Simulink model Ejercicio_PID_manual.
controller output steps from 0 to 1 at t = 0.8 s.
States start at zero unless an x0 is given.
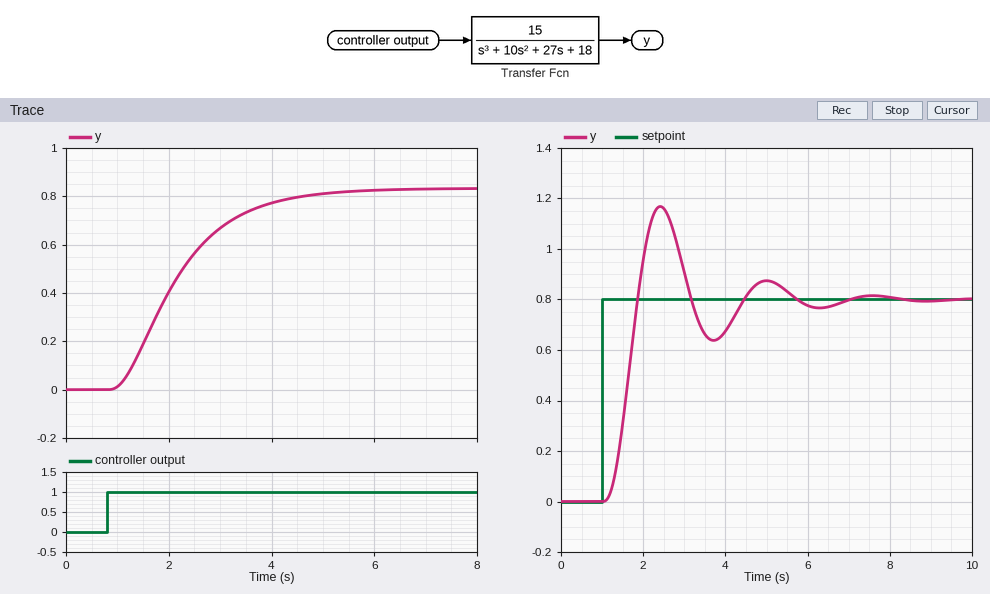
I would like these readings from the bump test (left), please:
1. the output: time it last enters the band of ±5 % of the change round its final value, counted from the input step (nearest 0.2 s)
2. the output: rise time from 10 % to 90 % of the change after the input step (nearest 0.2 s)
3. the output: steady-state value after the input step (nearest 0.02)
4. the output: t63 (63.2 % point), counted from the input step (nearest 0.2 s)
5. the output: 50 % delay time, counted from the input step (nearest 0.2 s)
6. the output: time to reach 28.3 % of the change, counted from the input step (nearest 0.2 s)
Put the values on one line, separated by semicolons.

3.6 s; 2.4 s; 0.84; 1.6 s; 1.2 s; 0.8 s
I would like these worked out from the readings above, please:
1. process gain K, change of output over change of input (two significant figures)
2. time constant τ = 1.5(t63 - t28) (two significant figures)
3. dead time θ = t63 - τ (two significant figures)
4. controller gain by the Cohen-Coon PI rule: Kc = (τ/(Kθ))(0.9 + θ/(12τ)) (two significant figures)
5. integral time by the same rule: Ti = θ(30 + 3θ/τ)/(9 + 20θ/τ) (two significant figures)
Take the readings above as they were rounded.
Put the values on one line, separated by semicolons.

0.84; 1.2 s; 0.40 s; 3.3; 0.79 s
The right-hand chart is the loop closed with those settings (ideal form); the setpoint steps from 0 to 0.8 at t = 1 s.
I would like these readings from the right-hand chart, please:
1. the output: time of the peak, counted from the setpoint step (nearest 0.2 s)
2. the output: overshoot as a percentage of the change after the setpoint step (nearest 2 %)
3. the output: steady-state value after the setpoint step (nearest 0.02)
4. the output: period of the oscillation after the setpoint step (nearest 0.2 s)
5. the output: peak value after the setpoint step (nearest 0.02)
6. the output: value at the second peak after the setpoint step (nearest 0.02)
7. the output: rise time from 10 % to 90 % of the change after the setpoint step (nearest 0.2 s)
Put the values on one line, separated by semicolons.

1.4 s; 46 %; 0.80; 2.6 s; 1.16; 0.88; 0.6 s
